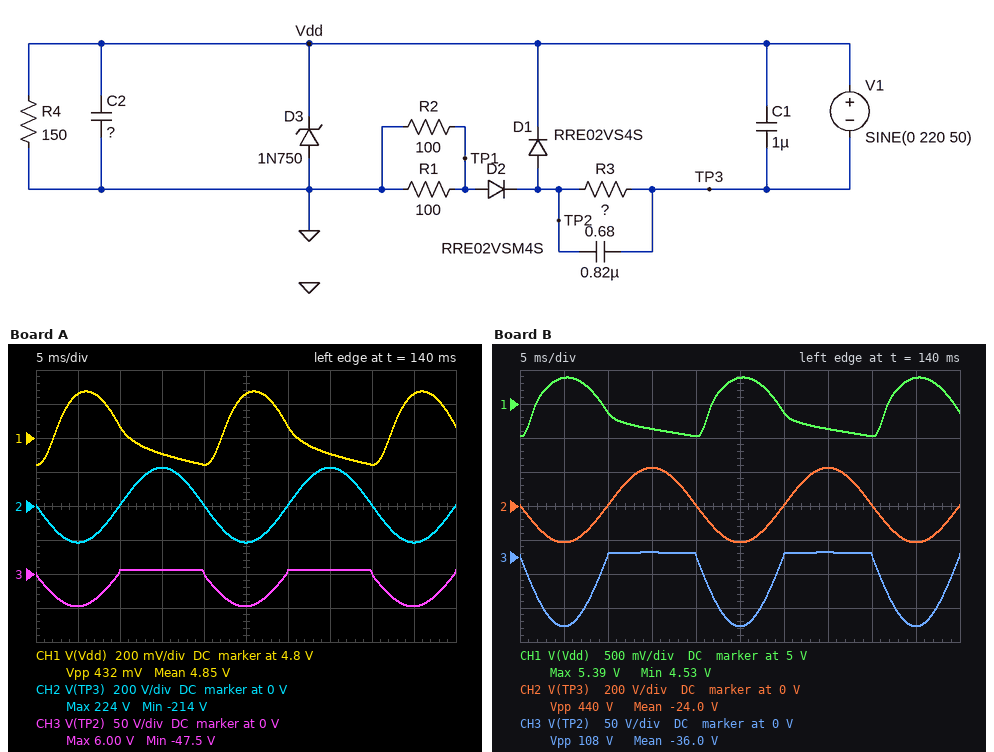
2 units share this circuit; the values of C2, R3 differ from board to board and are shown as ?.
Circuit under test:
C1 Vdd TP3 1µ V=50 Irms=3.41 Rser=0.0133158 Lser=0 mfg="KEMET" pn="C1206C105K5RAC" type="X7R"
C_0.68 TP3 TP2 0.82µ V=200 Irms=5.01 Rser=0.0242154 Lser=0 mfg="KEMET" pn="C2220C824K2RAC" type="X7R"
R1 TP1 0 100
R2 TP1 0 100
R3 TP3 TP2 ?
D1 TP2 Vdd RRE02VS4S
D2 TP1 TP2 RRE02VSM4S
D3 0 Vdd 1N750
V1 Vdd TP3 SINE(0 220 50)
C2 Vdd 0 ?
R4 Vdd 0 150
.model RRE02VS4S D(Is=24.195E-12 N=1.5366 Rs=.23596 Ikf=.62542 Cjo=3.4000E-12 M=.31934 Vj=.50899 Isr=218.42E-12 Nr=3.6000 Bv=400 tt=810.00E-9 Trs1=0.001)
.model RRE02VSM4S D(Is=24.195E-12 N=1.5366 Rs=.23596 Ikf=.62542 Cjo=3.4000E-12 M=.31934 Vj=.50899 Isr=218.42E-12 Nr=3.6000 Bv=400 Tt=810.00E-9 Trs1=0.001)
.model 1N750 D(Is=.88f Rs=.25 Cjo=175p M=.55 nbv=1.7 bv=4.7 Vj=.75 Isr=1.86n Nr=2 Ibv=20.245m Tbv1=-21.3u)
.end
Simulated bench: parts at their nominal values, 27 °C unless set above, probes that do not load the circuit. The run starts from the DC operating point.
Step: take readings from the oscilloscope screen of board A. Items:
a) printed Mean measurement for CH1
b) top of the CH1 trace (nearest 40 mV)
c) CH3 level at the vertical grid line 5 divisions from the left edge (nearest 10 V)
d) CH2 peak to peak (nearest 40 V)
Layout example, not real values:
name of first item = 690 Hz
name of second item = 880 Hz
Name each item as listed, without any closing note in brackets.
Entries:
printed Mean measurement for CH1 = 4.85 V
top of the CH1 trace = 5.08 V
CH3 level at the vertical grid line 5 divisions from the left edge = -50 V
CH2 peak to peak = 440 V
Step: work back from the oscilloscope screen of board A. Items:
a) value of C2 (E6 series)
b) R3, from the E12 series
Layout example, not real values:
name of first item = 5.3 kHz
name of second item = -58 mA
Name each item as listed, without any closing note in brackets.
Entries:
value of C2 = 3.3 mF
R3, from the E12 series = 180 Ω
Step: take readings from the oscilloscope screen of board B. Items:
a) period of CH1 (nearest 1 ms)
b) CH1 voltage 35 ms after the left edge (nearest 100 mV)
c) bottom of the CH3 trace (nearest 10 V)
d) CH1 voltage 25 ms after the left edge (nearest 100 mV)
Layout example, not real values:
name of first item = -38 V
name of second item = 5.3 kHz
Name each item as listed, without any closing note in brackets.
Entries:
period of CH1 = 20 ms
CH1 voltage 35 ms after the left edge = 4.6 V
bottom of the CH3 trace = -100 V
CH1 voltage 25 ms after the left edge = 5.4 V
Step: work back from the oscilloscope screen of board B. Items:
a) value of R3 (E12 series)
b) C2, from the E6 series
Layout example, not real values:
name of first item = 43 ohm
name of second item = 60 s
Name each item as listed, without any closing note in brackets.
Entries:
value of R3 = 56 Ω
C2, from the E6 series = 1.5 mF
